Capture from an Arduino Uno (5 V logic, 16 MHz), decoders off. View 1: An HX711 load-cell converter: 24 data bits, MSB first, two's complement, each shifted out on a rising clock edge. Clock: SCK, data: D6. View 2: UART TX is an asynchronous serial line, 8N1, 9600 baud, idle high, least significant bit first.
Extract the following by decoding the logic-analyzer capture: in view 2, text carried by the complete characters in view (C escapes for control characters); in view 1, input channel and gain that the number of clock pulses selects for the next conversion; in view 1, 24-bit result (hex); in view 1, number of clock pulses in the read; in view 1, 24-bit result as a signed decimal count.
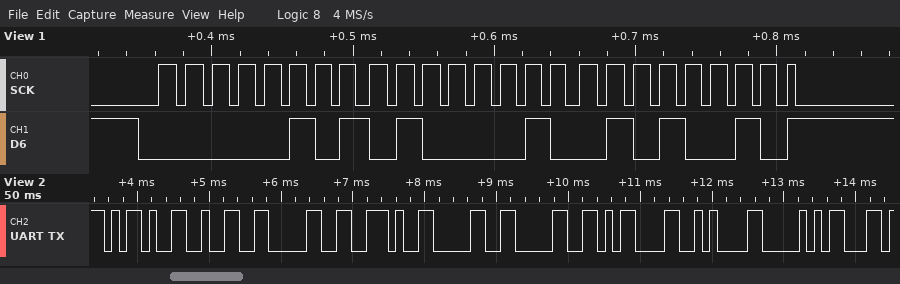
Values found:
"-20.00\r\nP"
channel A, gain 128
0x054252
25
344658
